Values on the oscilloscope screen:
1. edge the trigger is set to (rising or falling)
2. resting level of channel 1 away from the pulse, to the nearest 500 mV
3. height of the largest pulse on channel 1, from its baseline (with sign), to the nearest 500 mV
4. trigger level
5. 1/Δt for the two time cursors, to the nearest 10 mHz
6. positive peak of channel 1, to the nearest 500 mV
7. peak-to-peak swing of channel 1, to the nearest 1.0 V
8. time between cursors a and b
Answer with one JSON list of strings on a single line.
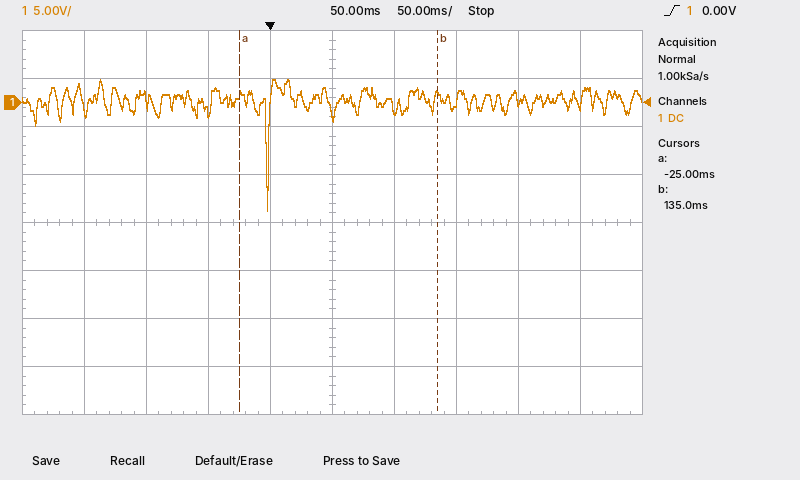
["rising", "500 mV", "-11.5 V", "0.00 V", "6.25 Hz", "2.5 V", "14.0 V", "160 ms"]
